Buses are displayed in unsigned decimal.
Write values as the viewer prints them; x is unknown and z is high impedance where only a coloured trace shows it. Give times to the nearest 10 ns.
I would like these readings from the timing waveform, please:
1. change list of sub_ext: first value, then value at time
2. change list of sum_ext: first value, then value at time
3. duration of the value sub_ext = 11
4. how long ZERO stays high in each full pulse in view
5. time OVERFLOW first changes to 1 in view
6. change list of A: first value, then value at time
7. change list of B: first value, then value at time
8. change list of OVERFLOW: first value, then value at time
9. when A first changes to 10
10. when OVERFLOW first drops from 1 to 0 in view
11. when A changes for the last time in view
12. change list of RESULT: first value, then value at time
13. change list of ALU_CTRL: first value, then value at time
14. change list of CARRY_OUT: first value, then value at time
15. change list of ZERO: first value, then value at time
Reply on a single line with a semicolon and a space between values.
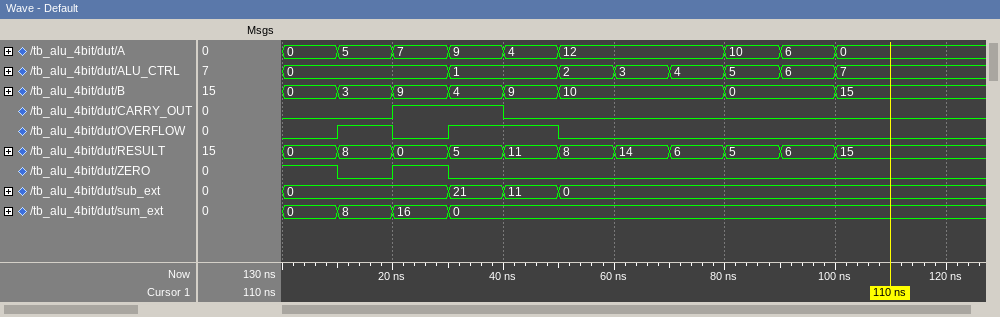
0, 21 at 30 ns, 11 at 40 ns, 0 at 50 ns; 0, 8 at 10 ns, 16 at 20 ns, 0 at 30 ns; 10 ns; 10 ns; 10 ns; 0, 5 at 10 ns, 7 at 20 ns, 9 at 30 ns, 4 at 40 ns, 12 at 50 ns, 10 at 80 ns, 6 at 90 ns, 0 at 100 ns; 0, 3 at 10 ns, 9 at 20 ns, 4 at 30 ns, 9 at 40 ns, 10 at 50 ns, 0 at 80 ns, 15 at 100 ns; 0, 1 at 10 ns, 0 at 20 ns, 1 at 30 ns, 0 at 50 ns; 80 ns; 20 ns; 100 ns; 0, 8 at 10 ns, 0 at 20 ns, 5 at 30 ns, 11 at 40 ns, 8 at 50 ns, 14 at 60 ns, 6 at 70 ns, 5 at 80 ns, 6 at 90 ns, 15 at 100 ns; 0, 1 at 30 ns, 2 at 50 ns, 3 at 60 ns, 4 at 70 ns, 5 at 80 ns, 6 at 90 ns, 7 at 100 ns; 0, 1 at 20 ns, 0 at 40 ns; 1, 0 at 10 ns, 1 at 20 ns, 0 at 30 ns
